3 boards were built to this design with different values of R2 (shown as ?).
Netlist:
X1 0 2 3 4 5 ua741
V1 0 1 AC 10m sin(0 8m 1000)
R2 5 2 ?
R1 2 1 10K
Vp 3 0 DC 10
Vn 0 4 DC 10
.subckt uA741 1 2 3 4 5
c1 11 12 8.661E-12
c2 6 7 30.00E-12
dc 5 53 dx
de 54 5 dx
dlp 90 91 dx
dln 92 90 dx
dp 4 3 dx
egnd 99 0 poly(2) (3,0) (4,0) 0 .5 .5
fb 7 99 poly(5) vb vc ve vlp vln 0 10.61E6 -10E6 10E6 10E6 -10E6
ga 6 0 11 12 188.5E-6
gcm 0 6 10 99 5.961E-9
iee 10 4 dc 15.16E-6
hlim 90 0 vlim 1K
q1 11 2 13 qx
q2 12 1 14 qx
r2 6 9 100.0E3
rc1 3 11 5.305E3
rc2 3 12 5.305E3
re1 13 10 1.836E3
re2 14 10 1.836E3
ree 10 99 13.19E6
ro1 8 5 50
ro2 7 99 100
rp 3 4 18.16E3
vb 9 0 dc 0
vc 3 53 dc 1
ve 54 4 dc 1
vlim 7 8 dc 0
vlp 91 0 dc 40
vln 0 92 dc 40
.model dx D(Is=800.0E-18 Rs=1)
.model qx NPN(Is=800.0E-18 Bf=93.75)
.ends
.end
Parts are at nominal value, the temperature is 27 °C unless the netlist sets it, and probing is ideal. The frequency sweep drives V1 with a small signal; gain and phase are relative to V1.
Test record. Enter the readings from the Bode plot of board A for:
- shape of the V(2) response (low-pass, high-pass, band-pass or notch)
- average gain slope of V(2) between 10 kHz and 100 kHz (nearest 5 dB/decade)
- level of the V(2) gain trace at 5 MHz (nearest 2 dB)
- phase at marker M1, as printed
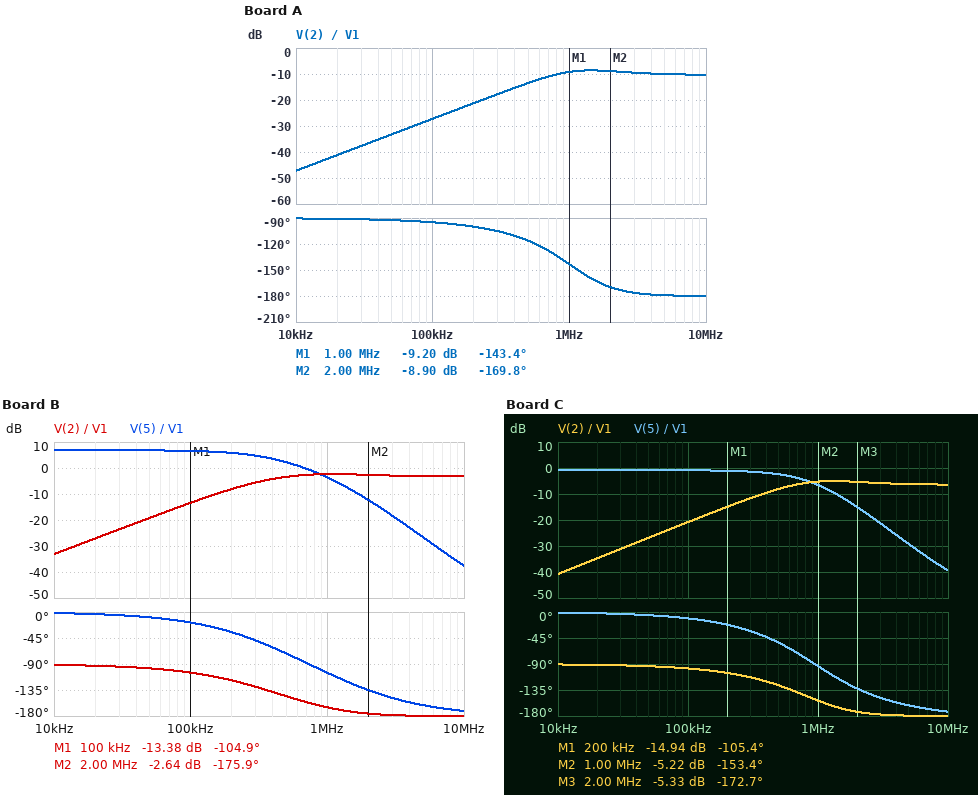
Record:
high-pass
20 dB/decade
-10 dB
-143.4 deg
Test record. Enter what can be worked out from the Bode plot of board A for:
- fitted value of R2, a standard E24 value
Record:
4.3 kΩ
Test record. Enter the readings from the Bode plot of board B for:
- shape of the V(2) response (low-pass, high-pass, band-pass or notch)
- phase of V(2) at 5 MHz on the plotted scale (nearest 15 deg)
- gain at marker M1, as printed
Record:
high-pass
-180 deg
-13.38 dB
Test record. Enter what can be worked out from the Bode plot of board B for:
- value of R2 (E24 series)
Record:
22 kΩ
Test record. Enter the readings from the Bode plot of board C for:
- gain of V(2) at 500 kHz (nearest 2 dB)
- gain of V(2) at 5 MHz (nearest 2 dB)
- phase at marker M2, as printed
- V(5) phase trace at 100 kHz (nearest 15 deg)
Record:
-8 dB
-6 dB
-153.4 deg
-15 deg
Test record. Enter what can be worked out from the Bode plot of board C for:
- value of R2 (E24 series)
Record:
9.1 kΩ
